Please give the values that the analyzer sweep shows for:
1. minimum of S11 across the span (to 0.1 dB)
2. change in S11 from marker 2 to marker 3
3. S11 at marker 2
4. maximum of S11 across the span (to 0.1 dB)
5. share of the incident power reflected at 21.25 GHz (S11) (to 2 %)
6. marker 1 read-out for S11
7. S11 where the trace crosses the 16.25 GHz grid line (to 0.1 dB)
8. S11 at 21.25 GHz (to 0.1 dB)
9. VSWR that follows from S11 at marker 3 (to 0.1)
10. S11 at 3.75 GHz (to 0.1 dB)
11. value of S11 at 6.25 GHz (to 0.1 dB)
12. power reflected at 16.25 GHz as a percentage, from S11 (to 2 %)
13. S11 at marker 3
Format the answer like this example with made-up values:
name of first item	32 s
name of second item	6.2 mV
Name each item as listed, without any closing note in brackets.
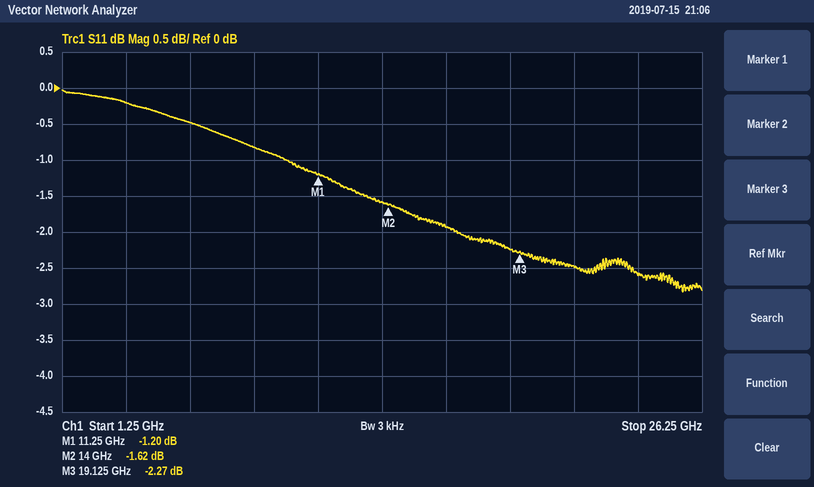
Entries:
minimum of S11 across the span	-2.8 dB
change in S11 from marker 2 to marker 3	-0.65 dB
S11 at marker 2	-1.62 dB
maximum of S11 across the span	0.0 dB
share of the incident power reflected at 21.25 GHz (S11)	56 %
marker 1 read-out for S11	-1.20 dB
S11 where the trace crosses the 16.25 GHz grid line	-1.9 dB
S11 at 21.25 GHz	-2.5 dB
VSWR that follows from S11 at marker 3	7.7
S11 at 3.75 GHz	-0.2 dB
value of S11 at 6.25 GHz	-0.5 dB
power reflected at 16.25 GHz as a percentage, from S11	64 %
S11 at marker 3	-2.27 dB
